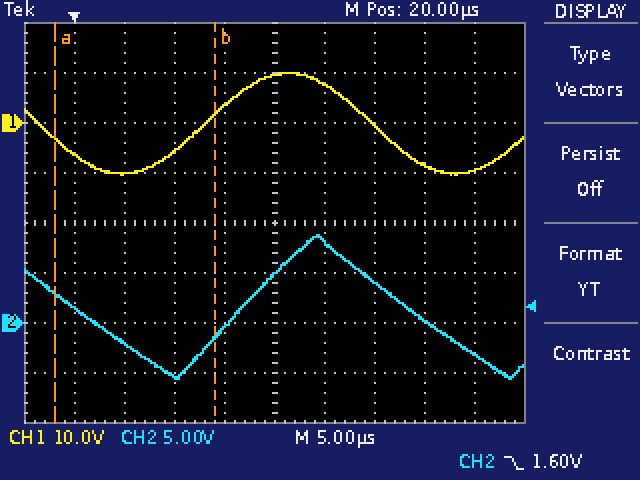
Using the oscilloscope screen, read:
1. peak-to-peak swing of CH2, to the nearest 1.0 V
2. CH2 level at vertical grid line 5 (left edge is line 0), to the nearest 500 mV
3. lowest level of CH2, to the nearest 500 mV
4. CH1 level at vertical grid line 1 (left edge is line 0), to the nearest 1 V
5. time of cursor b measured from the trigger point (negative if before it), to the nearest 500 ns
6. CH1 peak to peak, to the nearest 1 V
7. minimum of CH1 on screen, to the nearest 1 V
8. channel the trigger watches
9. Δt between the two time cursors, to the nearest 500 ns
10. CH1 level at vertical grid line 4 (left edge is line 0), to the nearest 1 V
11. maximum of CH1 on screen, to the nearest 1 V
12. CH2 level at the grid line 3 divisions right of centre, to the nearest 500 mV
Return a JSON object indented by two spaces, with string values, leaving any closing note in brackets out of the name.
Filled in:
{
  "peak-to-peak swing of CH2, to the nearest 1.0 V": "14.0 V",
  "CH2 level at vertical grid line 5 (left edge is line 0), to the nearest 500 mV": "5.0 V",
  "lowest level of CH2, to the nearest 500 mV": "-5.5 V",
  "CH1 level at vertical grid line 1 (left edge is line 0), to the nearest 1 V": "-6 V",
  "time of cursor b measured from the trigger point (negative if before it), to the nearest 500 ns": "+14.0 µs",
  "CH1 peak to peak, to the nearest 1 V": "20 V",
  "minimum of CH1 on screen, to the nearest 1 V": "-10 V",
  "channel the trigger watches": "CH2",
  "Δt between the two time cursors, to the nearest 500 ns": "16.0 µs",
  "CH1 level at vertical grid line 4 (left edge is line 0), to the nearest 1 V": "3 V",
  "maximum of CH1 on screen, to the nearest 1 V": "10 V",
  "CH2 level at the grid line 3 divisions right of centre, to the nearest 500 mV": "500 mV"
}
